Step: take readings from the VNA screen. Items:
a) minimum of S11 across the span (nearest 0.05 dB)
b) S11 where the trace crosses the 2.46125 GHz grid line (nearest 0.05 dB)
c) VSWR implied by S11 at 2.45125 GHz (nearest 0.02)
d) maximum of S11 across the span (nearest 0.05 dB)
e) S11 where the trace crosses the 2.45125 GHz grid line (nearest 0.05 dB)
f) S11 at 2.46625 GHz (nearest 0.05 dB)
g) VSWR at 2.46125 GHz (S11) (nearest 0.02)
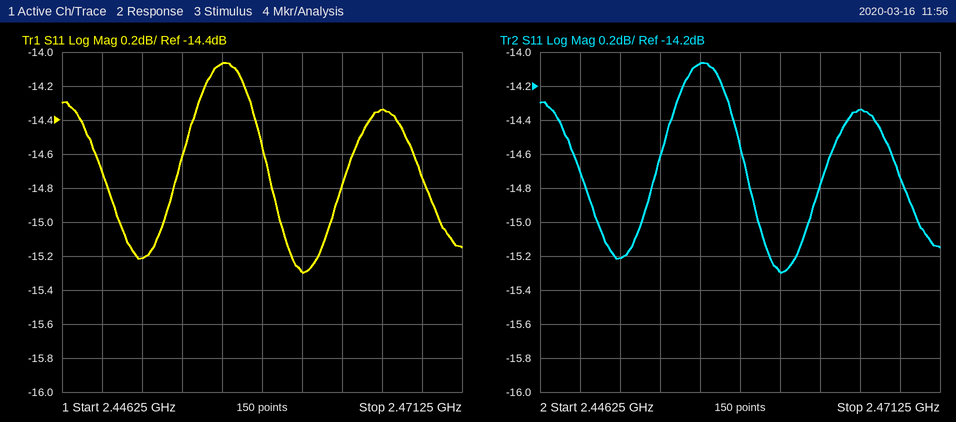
-15.30 dB
-15.30 dB
1.42
-14.05 dB
-15.20 dB
-14.35 dB
1.42
